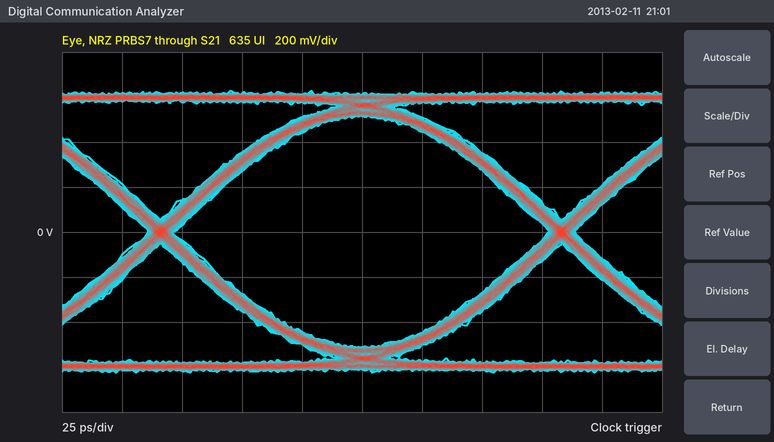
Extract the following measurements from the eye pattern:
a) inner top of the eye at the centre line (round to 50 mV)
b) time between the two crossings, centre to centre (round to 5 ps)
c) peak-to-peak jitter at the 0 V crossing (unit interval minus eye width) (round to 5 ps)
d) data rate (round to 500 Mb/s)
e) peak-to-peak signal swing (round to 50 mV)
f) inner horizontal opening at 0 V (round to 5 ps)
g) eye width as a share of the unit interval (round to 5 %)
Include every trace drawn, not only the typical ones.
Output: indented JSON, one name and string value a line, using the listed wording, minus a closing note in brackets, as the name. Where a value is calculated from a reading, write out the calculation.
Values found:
{
  "inner top of the eye at the centre line": "500 mV",
  "time between the two crossings, centre to centre": "165 ps",
  "peak-to-peak jitter at the 0 V crossing (unit interval minus eye width)": "10 ps",
  "data rate": "6.0 Gb/s",
  "peak-to-peak signal swing": "1.25 V",
  "inner horizontal opening at 0 V": "155 ps",
  "eye width as a share of the unit interval": "155 ps / 165 ps ≈ 93.9 %, so 95 % to the nearest 5 %"
}
